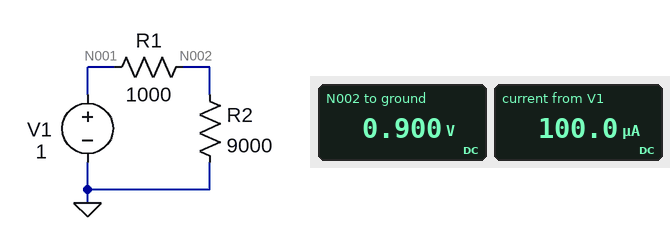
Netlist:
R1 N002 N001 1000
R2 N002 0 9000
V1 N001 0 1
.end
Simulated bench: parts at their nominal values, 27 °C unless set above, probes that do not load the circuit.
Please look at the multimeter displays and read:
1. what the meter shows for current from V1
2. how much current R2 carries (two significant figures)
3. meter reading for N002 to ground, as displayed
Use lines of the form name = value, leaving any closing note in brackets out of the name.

what the meter shows for current from V1 = 100.0 µA
how much current R2 carries = 100 µA
meter reading for N002 to ground, as displayed = 0.900 V
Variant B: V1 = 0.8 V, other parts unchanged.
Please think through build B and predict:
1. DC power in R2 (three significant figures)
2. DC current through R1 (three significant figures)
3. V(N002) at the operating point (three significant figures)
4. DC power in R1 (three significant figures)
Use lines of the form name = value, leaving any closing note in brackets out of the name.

DC power in R2 = 57.6 µW
DC current through R1 = 80.0 µA
V(N002) at the operating point = 720 mV
DC power in R1 = 6.40 µW
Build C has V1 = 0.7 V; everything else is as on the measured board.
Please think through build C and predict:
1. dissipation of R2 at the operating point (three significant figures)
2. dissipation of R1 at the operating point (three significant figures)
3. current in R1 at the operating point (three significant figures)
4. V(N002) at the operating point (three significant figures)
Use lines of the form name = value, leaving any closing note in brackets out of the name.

dissipation of R2 at the operating point = 44.1 µW
dissipation of R1 at the operating point = 4.90 µW
current in R1 at the operating point = 70.0 µA
V(N002) at the operating point = 630 mV
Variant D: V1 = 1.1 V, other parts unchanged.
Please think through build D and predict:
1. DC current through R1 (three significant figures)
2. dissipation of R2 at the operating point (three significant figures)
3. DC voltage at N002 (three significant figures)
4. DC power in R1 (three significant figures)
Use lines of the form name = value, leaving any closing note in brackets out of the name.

DC current through R1 = 110 µA
dissipation of R2 at the operating point = 109 µW
DC voltage at N002 = 990 mV
DC power in R1 = 12.1 µW
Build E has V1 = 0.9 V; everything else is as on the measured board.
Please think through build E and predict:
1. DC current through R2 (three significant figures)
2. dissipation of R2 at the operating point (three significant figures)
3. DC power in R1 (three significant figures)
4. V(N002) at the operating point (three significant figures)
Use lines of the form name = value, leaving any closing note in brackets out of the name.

DC current through R2 = 90.0 µA
dissipation of R2 at the operating point = 72.9 µW
DC power in R1 = 8.10 µW
V(N002) at the operating point = 810 mV
